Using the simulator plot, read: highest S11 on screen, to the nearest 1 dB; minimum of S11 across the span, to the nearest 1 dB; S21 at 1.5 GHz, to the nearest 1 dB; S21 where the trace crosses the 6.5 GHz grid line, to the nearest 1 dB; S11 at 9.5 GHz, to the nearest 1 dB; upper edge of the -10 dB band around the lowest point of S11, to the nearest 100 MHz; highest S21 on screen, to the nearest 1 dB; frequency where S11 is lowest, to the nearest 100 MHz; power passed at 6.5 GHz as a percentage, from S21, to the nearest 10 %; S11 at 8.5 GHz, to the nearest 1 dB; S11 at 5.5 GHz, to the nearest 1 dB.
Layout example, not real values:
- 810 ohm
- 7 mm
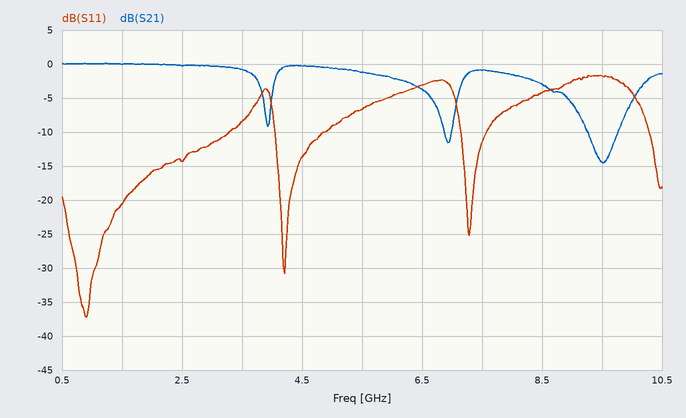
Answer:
- -2 dB
- -37 dB
- 0 dB
- -4 dB
- -2 dB
- 3.3 GHz
- 0 dB
- 900 MHz
- 40 %
- -4 dB
- -7 dB
